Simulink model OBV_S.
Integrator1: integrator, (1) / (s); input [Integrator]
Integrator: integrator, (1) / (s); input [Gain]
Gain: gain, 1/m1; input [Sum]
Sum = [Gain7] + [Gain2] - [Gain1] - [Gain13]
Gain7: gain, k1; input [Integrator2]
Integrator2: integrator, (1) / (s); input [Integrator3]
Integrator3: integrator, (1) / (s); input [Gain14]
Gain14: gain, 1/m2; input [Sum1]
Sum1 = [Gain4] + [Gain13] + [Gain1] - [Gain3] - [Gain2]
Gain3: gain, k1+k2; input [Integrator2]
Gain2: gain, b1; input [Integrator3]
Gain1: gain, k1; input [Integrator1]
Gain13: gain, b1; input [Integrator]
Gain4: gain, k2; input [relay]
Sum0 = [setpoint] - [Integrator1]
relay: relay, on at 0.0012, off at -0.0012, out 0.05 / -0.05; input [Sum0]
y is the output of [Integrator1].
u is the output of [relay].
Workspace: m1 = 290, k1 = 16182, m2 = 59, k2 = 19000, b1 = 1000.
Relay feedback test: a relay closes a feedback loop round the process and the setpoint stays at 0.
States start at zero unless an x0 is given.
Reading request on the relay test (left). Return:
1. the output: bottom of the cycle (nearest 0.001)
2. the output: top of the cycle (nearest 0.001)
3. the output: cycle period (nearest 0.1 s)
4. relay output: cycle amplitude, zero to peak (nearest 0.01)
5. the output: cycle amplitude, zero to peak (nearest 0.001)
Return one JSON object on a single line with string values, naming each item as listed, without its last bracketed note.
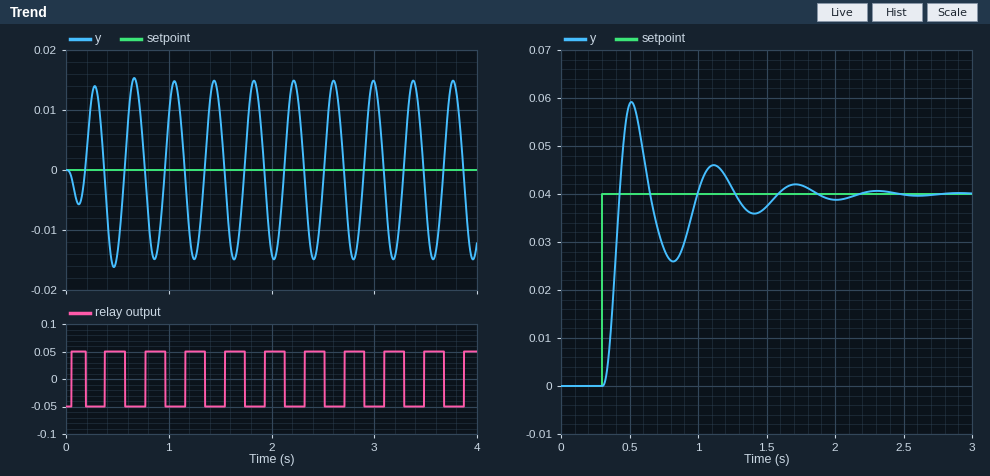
{"the output: bottom of the cycle": "-0.015", "the output: top of the cycle": "0.015", "the output: cycle period": "0.4 s", "relay output: cycle amplitude, zero to peak": "0.05", "the output: cycle amplitude, zero to peak": "0.015"}
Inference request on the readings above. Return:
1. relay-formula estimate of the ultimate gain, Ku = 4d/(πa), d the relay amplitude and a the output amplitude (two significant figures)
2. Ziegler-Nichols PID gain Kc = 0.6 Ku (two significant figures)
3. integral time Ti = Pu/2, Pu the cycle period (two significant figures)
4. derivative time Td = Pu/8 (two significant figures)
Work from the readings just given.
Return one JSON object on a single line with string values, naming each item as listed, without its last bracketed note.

{"relay-formula estimate of the ultimate gain, Ku = 4d/(πa), d the relay amplitude and a the output amplitude": "4.2", "Ziegler-Nichols PID gain Kc = 0.6 Ku": "2.5", "integral time Ti = Pu/2, Pu the cycle period": "0.20 s", "derivative time Td = Pu/8": "0.050 s"}
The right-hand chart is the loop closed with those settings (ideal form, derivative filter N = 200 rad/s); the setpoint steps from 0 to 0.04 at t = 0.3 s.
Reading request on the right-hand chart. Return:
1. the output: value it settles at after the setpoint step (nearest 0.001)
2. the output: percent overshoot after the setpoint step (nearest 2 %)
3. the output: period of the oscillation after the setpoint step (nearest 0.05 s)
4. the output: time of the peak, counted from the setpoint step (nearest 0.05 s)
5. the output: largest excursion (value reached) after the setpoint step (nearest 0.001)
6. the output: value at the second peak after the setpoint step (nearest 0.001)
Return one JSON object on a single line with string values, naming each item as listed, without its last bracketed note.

{"the output: value it settles at after the setpoint step": "0.040", "the output: percent overshoot after the setpoint step": "48 %", "the output: period of the oscillation after the setpoint step": "0.60 s", "the output: time of the peak, counted from the setpoint step": "0.20 s", "the output: largest excursion (value reached) after the setpoint step": "0.059", "the output: value at the second peak after the setpoint step": "0.046"}
